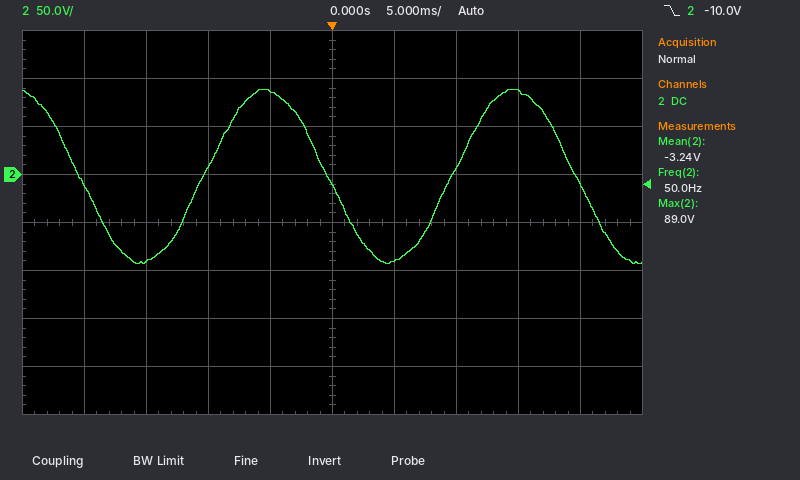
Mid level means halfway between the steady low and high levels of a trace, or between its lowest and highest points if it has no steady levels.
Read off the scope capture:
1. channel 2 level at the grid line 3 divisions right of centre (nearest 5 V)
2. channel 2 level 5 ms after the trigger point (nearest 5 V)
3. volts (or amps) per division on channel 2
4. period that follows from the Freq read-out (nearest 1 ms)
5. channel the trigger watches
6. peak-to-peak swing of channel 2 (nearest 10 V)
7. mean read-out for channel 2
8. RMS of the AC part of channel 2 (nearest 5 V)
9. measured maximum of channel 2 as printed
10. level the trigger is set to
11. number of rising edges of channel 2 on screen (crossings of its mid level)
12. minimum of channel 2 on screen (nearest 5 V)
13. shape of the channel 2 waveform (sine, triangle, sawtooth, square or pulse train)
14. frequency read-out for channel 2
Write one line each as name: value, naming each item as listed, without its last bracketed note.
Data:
channel 2 level at the grid line 3 divisions right of centre: 85 V
channel 2 level 5 ms after the trigger point: -90 V
volts (or amps) per division on channel 2: 50 V
period that follows from the Freq read-out: 20 ms
channel the trigger watches: channel 2
peak-to-peak swing of channel 2: 180 V
mean read-out for channel 2: -3.24 V
RMS of the AC part of channel 2: 65 V
measured maximum of channel 2 as printed: 89.0 V
level the trigger is set to: -10.0 V
number of rising edges of channel 2 on screen: 2
minimum of channel 2 on screen: -95 V
shape of the channel 2 waveform: sine
frequency read-out for channel 2: 50.0 Hz
